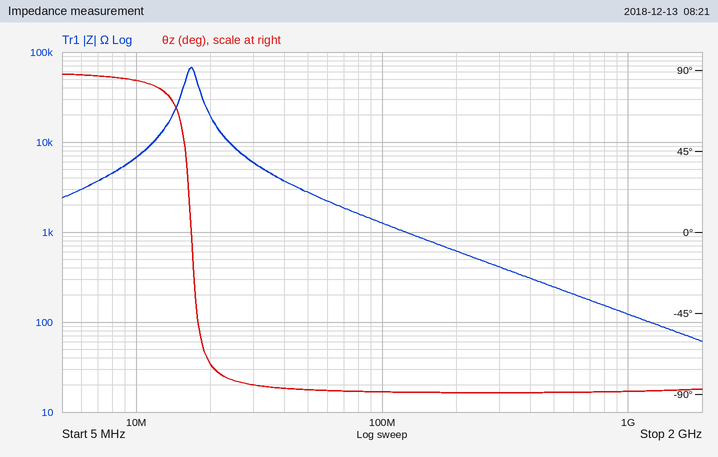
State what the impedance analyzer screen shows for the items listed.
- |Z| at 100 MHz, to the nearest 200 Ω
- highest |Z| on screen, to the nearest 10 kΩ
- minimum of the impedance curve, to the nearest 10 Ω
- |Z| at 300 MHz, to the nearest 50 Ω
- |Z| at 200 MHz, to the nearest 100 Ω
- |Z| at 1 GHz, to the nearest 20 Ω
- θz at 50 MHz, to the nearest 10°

1.2 kΩ
70 kΩ
60 Ω
400 Ω
600 Ω
120 Ω
-90°
